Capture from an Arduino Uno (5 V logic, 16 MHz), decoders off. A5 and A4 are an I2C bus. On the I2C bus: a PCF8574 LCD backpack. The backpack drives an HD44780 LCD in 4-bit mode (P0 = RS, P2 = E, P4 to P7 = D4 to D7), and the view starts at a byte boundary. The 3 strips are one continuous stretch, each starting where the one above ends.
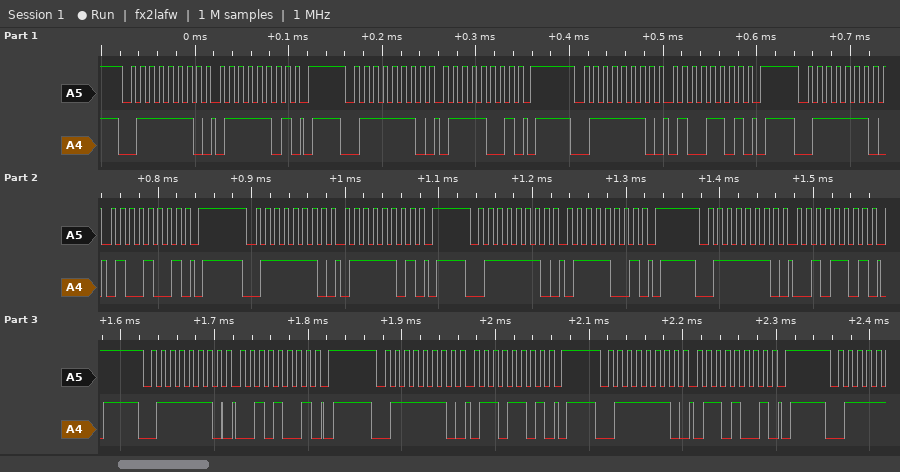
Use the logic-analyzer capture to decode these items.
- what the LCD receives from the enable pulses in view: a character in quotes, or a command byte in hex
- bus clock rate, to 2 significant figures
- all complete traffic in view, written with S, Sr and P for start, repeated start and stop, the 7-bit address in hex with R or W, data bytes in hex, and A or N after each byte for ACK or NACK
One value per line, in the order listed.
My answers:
't' 'r'
100 kHz
S 3FW A 7D A P S 3FW A 79 A P S 3FW A 4D A P S 3FW A 49 A P S 3FW A 7D A P S 3FW A 79 A P S 3FW A 2D A P S 3FW A 29 A P S 3FW A 6D A P S 3FW A 69 A P
